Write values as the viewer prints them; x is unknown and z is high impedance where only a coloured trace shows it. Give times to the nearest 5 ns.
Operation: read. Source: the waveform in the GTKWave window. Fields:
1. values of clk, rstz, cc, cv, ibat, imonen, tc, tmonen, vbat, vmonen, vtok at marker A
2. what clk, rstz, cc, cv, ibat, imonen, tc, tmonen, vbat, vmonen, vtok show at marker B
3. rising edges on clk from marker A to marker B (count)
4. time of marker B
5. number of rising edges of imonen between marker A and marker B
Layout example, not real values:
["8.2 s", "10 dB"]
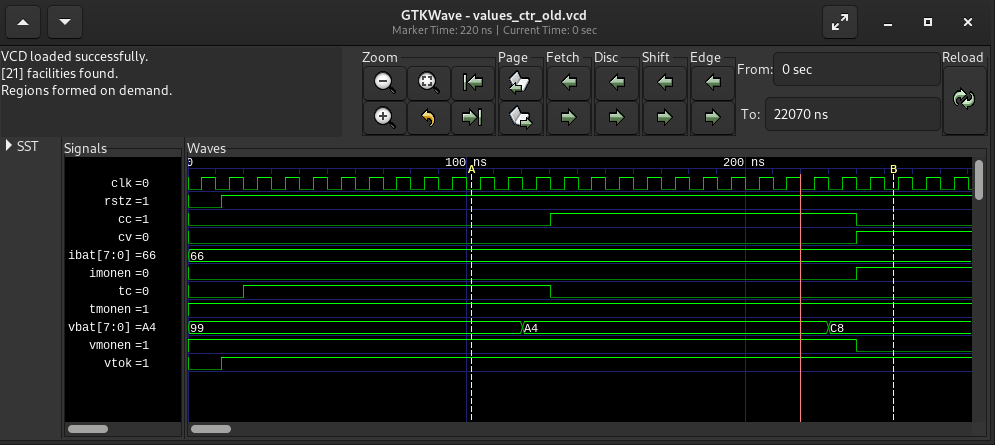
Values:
["clk=0, rstz=1, cc=0, cv=0, ibat=66, imonen=0, tc=1, tmonen=1, vbat=99, vmonen=1, vtok=1", "clk=0, rstz=1, cc=0, cv=1, ibat=66, imonen=1, tc=0, tmonen=1, vbat=C8, vmonen=0, vtok=1", "15", "255 ns", "1"]
